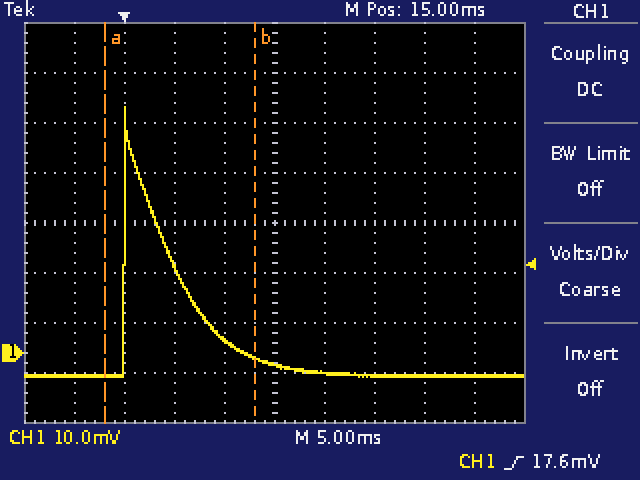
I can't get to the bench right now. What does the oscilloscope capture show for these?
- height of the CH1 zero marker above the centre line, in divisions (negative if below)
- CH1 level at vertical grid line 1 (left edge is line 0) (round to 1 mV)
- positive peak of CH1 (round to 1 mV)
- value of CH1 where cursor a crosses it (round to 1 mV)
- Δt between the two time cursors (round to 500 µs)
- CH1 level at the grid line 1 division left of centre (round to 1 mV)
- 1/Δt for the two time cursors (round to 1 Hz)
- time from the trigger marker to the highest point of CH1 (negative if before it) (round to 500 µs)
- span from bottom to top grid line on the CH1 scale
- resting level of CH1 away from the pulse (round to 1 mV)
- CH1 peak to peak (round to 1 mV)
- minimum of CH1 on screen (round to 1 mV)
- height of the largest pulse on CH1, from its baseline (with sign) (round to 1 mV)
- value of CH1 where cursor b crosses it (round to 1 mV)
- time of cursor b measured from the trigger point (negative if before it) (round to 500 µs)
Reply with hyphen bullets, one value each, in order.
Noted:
- -2.6 div
- -5 mV
- 49 mV
- -5 mV
- 15.0 ms
- 3 mV
- 67 Hz
- 0.0 ms
- 80 mV
- -5 mV
- 54 mV
- -5 mV
- +54 mV
- -1 mV
- +13.0 ms
